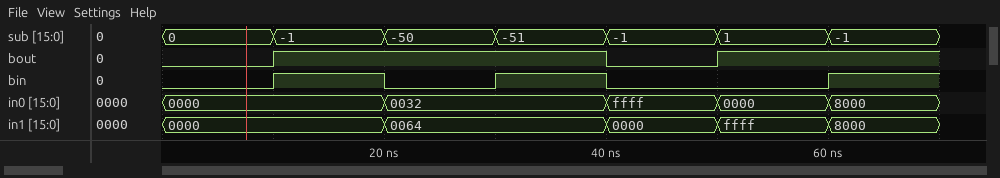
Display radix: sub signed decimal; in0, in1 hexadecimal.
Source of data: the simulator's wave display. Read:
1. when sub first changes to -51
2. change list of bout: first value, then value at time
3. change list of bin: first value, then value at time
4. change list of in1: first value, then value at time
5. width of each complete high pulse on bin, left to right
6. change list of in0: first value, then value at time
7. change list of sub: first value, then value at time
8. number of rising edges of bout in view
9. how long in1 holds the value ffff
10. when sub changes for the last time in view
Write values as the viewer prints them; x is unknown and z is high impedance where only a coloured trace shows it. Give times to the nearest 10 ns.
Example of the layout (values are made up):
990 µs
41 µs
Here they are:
30 ns
0, 1 at 10 ns, 0 at 40 ns, 1 at 50 ns
0, 1 at 10 ns, 0 at 20 ns, 1 at 30 ns, 0 at 40 ns, 1 at 60 ns
0000, 0064 at 20 ns, 0000 at 40 ns, ffff at 50 ns, 8000 at 60 ns
10 ns, 10 ns
0000, 0032 at 20 ns, ffff at 40 ns, 0000 at 50 ns, 8000 at 60 ns
0, -1 at 10 ns, -50 at 20 ns, -51 at 30 ns, -1 at 40 ns, 1 at 50 ns, -1 at 60 ns
2
10 ns
60 ns
